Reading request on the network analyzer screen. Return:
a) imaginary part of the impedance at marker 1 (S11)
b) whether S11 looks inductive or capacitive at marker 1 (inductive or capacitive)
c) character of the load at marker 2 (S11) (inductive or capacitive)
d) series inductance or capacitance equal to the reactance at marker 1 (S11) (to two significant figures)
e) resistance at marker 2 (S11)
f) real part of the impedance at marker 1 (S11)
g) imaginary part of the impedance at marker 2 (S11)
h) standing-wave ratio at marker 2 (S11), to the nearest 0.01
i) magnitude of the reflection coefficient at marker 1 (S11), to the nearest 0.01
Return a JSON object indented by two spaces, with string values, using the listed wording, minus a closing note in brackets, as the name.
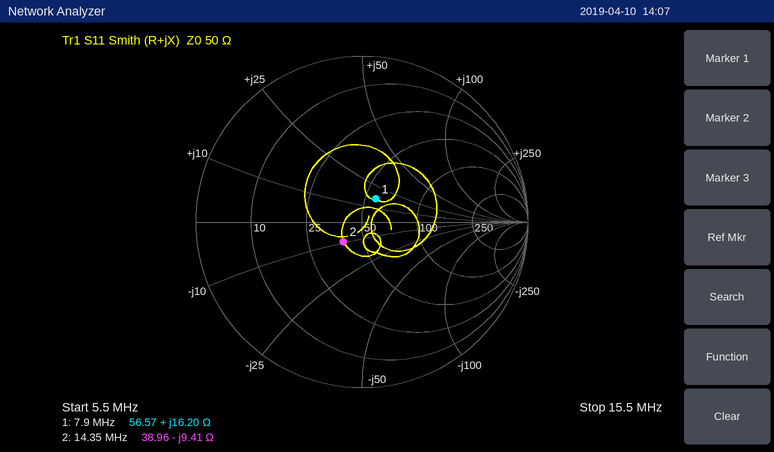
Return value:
{
  "imaginary part of the impedance at marker 1": "+16.20 Ω",
  "whether S11 looks inductive or capacitive at marker 1": "inductive",
  "character of the load at marker 2 (S11)": "capacitive",
  "series inductance or capacitance equal to the reactance at marker 1 (S11)": "330 nH",
  "resistance at marker 2": "38.96 Ω",
  "real part of the impedance at marker 1": "56.57 Ω",
  "imaginary part of the impedance at marker 2": "-9.41 Ω",
  "standing-wave ratio at marker 2 (S11), to the nearest 0.01": "1.39",
  "magnitude of the reflection coefficient at marker 1 (S11), to the nearest 0.01": "0.16"
}
